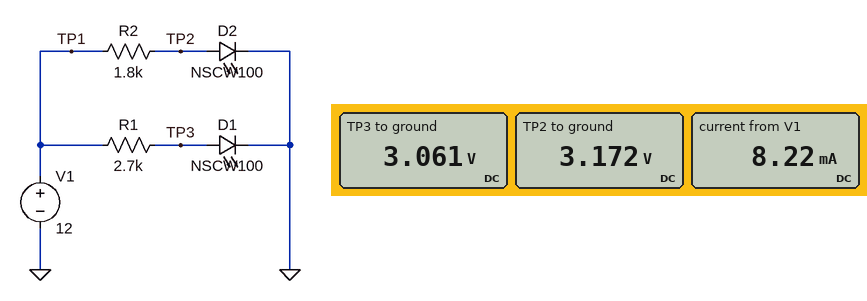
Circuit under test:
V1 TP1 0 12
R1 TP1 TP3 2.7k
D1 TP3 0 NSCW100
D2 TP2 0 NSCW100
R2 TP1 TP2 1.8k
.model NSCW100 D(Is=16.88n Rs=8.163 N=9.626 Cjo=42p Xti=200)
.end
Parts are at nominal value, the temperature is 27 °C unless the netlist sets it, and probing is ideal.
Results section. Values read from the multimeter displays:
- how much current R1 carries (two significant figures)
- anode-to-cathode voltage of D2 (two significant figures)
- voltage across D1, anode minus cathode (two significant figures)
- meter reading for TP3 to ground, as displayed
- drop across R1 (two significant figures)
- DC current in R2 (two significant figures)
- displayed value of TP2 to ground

3.3 mA
3.2 V
3.1 V
3.061 V
8.9 V
4.9 mA
3.172 V
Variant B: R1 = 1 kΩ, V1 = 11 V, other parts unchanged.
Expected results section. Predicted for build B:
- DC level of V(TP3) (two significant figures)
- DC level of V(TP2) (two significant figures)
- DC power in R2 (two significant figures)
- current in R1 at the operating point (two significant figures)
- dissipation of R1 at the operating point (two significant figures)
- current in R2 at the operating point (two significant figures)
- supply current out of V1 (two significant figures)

3.3 V
3.1 V
34 mW
7.7 mA
59 mW
4.4 mA
12 mA
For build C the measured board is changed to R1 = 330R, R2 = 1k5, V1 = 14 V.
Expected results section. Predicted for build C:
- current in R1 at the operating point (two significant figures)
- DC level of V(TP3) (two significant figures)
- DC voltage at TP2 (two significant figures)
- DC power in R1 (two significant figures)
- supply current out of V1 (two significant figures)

31 mA
3.8 V
3.3 V
310 mW
38 mA
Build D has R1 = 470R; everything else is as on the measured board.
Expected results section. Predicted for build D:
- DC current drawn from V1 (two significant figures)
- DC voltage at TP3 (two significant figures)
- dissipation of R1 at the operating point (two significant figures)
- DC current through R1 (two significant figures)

23 mA
3.6 V
150 mW
18 mA
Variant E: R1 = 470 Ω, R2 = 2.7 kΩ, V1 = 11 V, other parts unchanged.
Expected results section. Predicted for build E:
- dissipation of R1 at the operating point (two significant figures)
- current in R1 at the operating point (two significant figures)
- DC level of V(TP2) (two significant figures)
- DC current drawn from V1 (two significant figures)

120 mW
16 mA
3.0 V
19 mA
